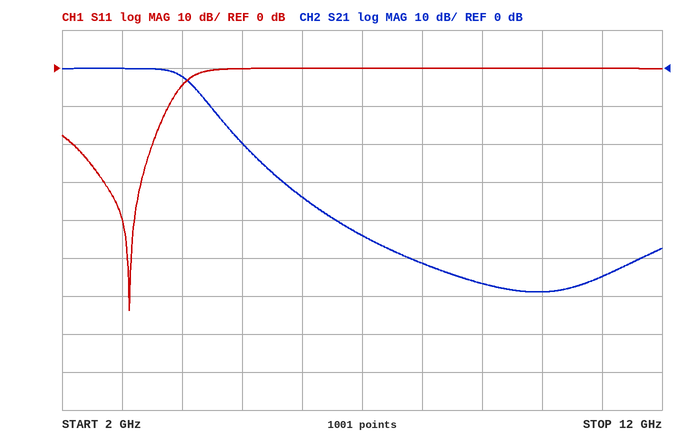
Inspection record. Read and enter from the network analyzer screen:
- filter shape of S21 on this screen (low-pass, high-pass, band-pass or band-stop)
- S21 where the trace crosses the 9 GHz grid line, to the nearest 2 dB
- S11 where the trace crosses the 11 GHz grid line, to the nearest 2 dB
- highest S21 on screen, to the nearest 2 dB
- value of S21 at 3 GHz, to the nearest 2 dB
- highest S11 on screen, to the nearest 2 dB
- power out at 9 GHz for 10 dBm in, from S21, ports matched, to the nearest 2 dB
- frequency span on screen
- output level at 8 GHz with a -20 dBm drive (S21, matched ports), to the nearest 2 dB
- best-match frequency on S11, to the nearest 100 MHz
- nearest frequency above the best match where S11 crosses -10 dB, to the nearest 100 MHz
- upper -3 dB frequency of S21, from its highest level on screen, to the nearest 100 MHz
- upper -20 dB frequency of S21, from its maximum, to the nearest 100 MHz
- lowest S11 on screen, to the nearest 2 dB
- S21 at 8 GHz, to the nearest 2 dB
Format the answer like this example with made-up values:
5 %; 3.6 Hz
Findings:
low-pass; -56 dB; 0 dB; 0 dB; 0 dB; 0 dB; -46 dBm; 10 GHz; -72 dBm; 3.1 GHz; 3.8 GHz; 4.1 GHz; 5.0 GHz; -64 dB; -52 dB
